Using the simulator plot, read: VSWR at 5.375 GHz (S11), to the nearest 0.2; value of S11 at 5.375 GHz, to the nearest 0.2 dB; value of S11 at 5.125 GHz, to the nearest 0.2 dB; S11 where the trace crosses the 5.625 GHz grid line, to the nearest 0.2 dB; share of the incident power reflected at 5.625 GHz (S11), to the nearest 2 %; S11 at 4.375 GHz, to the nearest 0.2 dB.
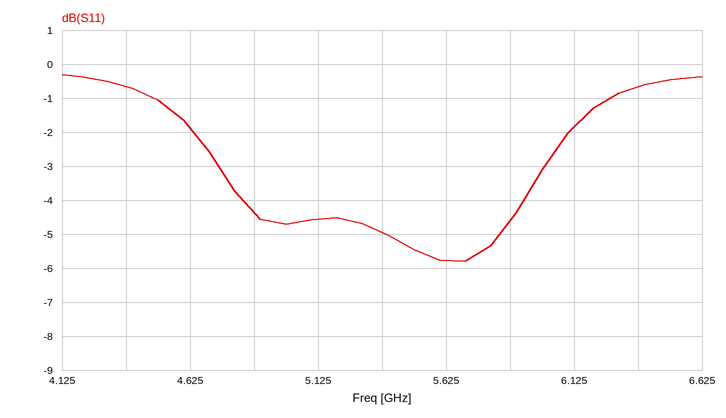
3.6
-5.0 dB
-4.6 dB
-5.8 dB
26 %
-0.6 dB
